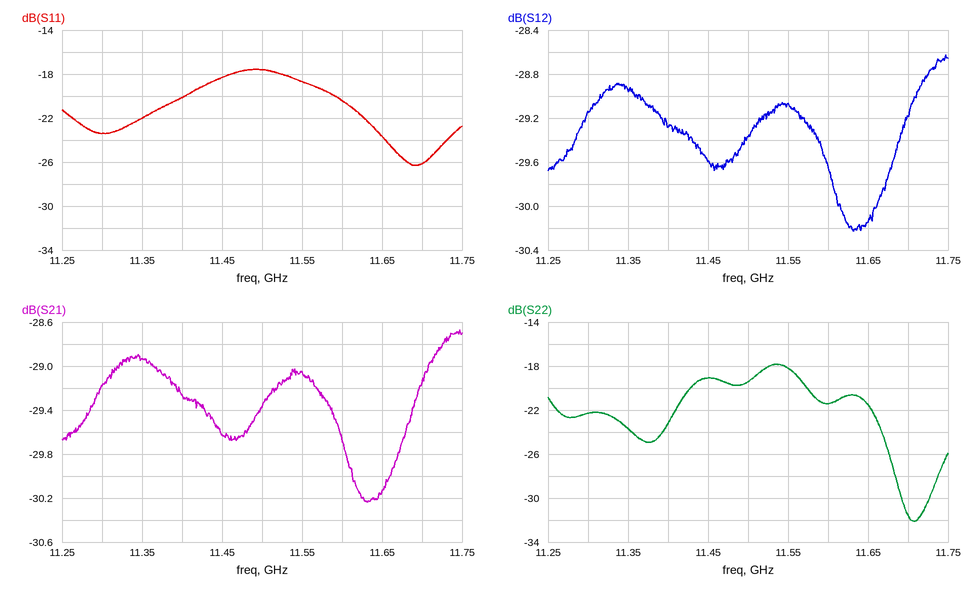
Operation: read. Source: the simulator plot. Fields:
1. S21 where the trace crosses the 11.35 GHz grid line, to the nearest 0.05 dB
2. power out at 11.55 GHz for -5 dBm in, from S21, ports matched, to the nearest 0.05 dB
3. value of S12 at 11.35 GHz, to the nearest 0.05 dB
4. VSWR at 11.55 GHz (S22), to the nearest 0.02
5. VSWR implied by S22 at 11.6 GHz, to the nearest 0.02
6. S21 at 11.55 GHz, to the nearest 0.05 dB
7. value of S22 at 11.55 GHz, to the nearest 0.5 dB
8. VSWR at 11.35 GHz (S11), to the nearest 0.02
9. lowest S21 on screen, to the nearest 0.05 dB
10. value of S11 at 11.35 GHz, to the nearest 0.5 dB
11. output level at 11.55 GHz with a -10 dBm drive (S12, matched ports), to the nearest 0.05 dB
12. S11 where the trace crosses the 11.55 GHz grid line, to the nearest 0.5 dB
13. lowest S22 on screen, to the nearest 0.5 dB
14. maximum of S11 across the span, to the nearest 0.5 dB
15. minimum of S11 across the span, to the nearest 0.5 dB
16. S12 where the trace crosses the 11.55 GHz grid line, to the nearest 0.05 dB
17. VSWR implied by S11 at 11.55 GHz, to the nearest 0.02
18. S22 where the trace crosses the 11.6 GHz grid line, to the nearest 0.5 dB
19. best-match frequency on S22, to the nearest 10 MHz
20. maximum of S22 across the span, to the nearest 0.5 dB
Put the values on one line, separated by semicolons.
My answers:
-28.95 dB; -34.05 dBm; -28.95 dB; 1.28; 1.18; -29.05 dB; -18.0 dB; 1.18; -30.25 dB; -22.0 dB; -39.05 dBm; -18.5 dB; -32.0 dB; -17.5 dB; -26.5 dB; -29.05 dB; 1.26; -21.5 dB; 11.71 GHz; -18.0 dB
